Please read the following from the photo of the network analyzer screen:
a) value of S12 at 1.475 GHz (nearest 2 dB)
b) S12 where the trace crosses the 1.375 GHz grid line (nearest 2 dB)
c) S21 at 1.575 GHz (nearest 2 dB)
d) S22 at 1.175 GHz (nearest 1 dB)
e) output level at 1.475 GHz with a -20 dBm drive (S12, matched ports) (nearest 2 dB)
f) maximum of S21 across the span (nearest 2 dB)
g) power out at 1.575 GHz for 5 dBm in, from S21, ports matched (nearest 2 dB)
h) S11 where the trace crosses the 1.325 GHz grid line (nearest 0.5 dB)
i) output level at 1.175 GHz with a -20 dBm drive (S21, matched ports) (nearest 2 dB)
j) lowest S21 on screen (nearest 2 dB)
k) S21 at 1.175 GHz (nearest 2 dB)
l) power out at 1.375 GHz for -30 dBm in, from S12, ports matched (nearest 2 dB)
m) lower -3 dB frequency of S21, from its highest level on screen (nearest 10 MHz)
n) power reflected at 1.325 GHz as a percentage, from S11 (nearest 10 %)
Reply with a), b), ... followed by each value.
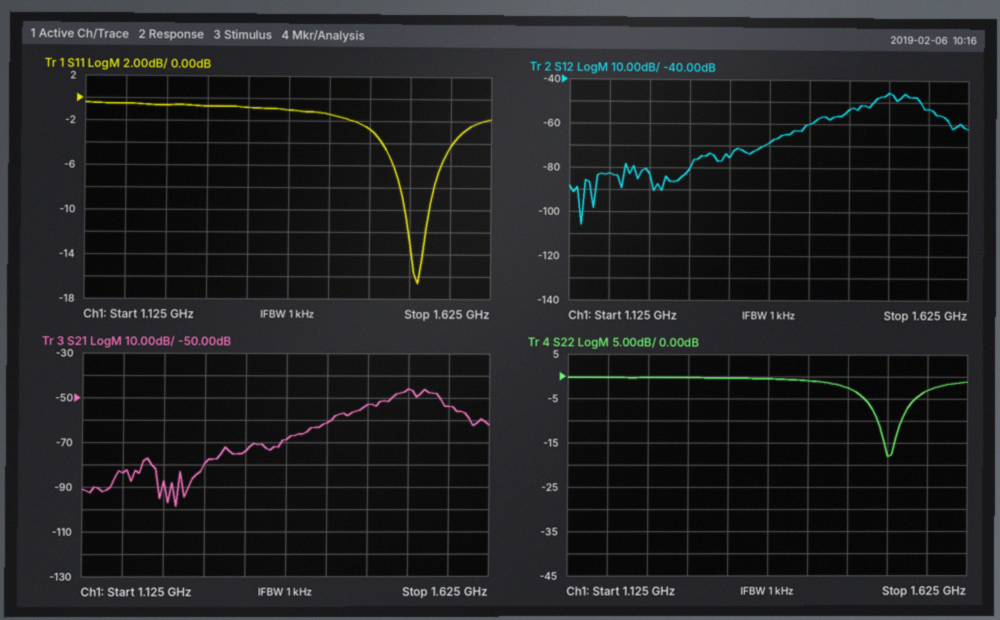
a) -54 dB
b) -68 dB
c) -54 dB
d) 0 dB
e) -74 dBm
f) -46 dB
g) -48 dBm
h) -1.0 dB
i) -104 dBm
j) -98 dB
k) -84 dB
l) -98 dBm
m) 1.51 GHz
n) 80 %
